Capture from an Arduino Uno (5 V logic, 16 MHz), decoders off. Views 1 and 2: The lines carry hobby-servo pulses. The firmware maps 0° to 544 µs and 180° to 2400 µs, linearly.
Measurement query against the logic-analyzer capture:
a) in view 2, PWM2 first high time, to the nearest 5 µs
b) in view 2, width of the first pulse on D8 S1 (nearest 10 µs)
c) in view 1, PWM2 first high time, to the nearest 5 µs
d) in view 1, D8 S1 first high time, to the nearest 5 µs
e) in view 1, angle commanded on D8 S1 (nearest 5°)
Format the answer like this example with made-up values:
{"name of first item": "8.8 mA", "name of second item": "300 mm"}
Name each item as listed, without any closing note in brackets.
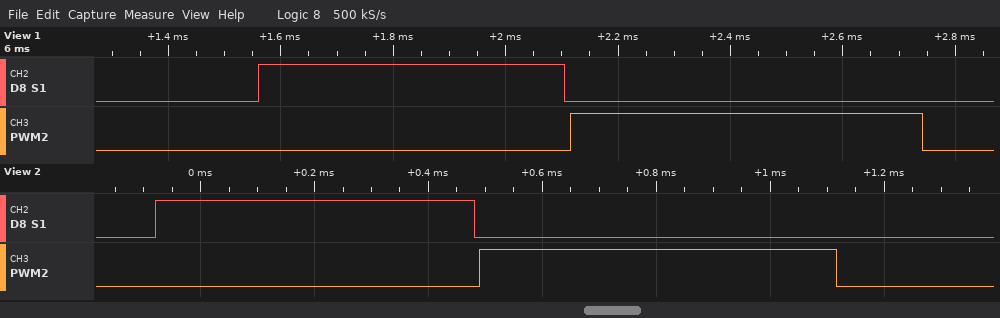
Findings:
{"in view 2, PWM2 first high time, to the nearest 5 µs": "625 µs", "in view 2, width of the first pulse on D8 S1": "560 µs", "in view 1, PWM2 first high time, to the nearest 5 µs": "625 µs", "in view 1, D8 S1 first high time, to the nearest 5 µs": "545 µs", "in view 1, angle commanded on D8 S1": "0°"}
